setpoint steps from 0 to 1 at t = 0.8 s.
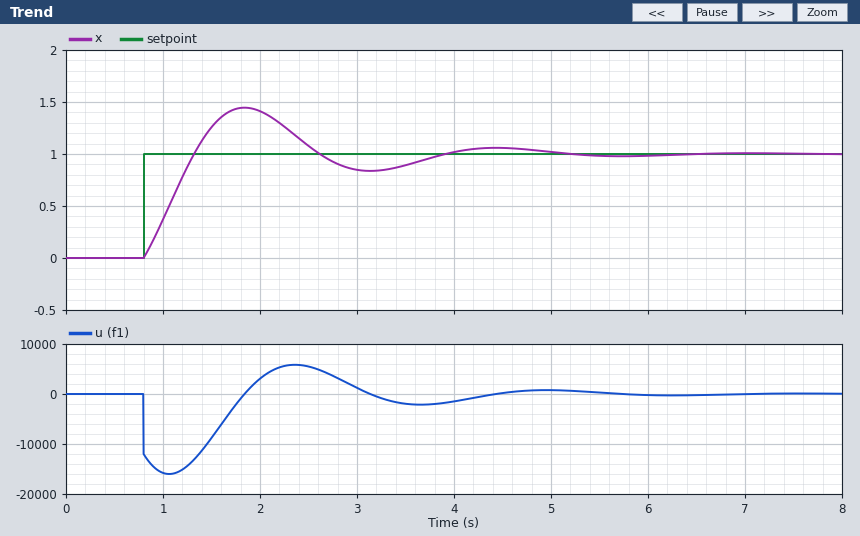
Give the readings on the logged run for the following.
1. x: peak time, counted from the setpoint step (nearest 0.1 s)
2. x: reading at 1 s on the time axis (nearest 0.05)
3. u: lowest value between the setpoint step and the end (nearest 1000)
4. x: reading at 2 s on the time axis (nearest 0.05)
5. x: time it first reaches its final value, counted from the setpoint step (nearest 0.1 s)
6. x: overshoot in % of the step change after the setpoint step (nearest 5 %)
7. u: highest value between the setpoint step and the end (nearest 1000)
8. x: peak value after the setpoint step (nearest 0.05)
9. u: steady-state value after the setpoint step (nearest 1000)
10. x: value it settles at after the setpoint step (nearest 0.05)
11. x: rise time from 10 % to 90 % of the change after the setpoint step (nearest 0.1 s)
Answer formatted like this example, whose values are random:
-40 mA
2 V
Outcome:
1.0 s
0.35
-16000
1.40
0.5 s
45 %
6000
1.45
0
1.00
0.4 s
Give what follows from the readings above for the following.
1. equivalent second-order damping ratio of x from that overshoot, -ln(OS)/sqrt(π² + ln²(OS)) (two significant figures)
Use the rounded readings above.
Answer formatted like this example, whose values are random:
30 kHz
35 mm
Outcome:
0.25
